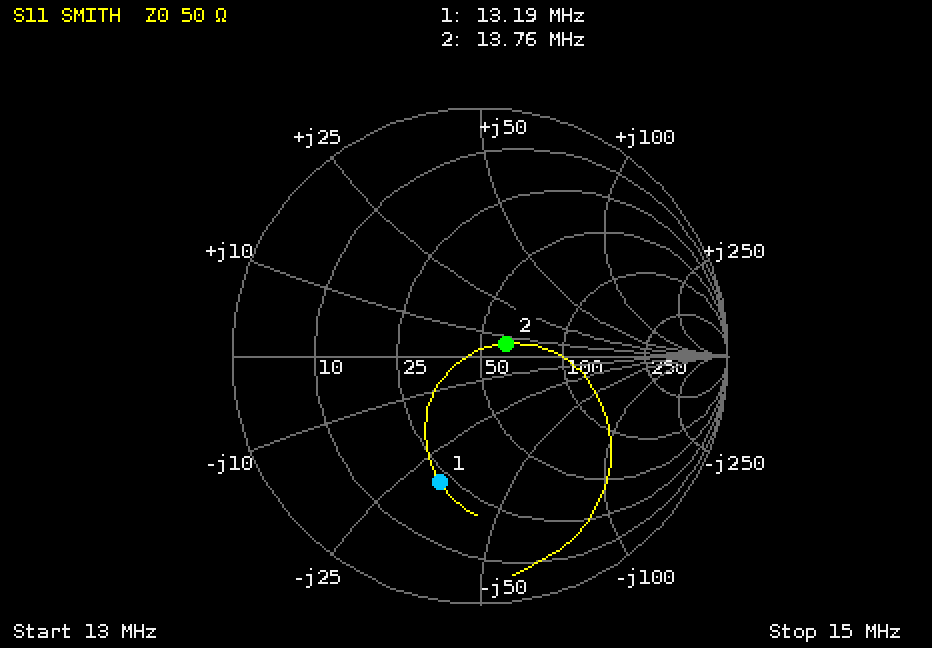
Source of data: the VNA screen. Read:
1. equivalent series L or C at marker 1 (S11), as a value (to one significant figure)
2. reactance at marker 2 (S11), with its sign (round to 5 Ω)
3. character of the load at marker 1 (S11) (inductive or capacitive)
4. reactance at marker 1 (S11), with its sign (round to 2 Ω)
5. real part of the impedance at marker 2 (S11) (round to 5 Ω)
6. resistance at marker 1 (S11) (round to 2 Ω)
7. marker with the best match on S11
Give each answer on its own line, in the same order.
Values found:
400 pF
+5 Ω
capacitive
-32 Ω
60 Ω
22 Ω
marker 2
